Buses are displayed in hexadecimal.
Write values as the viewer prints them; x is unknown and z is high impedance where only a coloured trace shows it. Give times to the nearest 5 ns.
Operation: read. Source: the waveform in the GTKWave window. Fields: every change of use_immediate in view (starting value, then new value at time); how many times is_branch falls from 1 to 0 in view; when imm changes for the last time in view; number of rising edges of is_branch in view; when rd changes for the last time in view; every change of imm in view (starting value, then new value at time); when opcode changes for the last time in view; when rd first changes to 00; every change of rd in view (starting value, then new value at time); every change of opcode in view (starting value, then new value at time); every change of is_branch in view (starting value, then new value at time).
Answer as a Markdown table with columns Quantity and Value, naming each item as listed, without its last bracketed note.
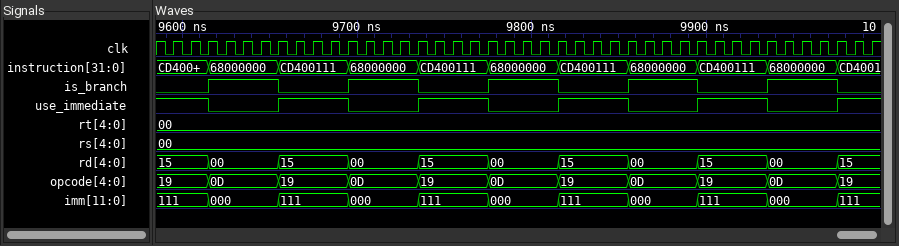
| Quantity | Value |
|---|---|
| every change of use_immediate in view | 1, 0 at 9615 ns, 1 at 9655 ns, 0 at 9695 ns, 1 at 9735 ns, 0 at 9775 ns, 1 at 9815 ns, 0 at 9855 ns, 1 at 9895 ns, 0 at 9935 ns, 1 at 9975 ns |
| how many times is_branch falls from 1 to 0 in view | 5 |
| when imm changes for the last time in view | 9975 ns |
| number of rising edges of is_branch in view | 5 |
| when rd changes for the last time in view | 9975 ns |
| every change of imm in view | 111, 000 at 9615 ns, 111 at 9655 ns, 000 at 9695 ns, 111 at 9735 ns, 000 at 9775 ns, 111 at 9815 ns, 000 at 9855 ns, 111 at 9895 ns, 000 at 9935 ns, 111 at 9975 ns |
| when opcode changes for the last time in view | 9975 ns |
| when rd first changes to 00 | 9615 ns |
| every change of rd in view | 15, 00 at 9615 ns, 15 at 9655 ns, 00 at 9695 ns, 15 at 9735 ns, 00 at 9775 ns, 15 at 9815 ns, 00 at 9855 ns, 15 at 9895 ns, 00 at 9935 ns, 15 at 9975 ns |
| every change of opcode in view | 19, 0D at 9615 ns, 19 at 9655 ns, 0D at 9695 ns, 19 at 9735 ns, 0D at 9775 ns, 19 at 9815 ns, 0D at 9855 ns, 19 at 9895 ns, 0D at 9935 ns, 19 at 9975 ns |
| every change of is_branch in view | 0, 1 at 9615 ns, 0 at 9655 ns, 1 at 9695 ns, 0 at 9735 ns, 1 at 9775 ns, 0 at 9815 ns, 1 at 9855 ns, 0 at 9895 ns, 1 at 9935 ns, 0 at 9975 ns |
